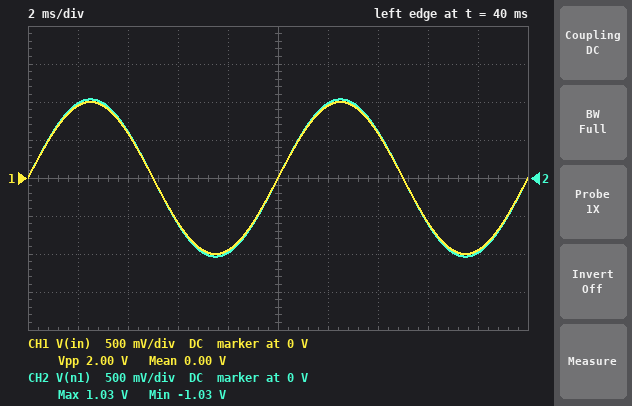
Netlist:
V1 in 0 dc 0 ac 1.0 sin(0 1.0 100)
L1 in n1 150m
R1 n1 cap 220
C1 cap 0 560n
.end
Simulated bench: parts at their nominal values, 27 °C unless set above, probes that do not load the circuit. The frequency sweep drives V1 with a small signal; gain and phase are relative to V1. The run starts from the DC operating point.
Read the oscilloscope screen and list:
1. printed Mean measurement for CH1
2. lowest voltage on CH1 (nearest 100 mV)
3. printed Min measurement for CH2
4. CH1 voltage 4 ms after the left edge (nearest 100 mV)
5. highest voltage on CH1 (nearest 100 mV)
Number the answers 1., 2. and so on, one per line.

1. 0.00 V
2. -1.0 V
3. -1.03 V
4. 600 mV
5. 1.0 V
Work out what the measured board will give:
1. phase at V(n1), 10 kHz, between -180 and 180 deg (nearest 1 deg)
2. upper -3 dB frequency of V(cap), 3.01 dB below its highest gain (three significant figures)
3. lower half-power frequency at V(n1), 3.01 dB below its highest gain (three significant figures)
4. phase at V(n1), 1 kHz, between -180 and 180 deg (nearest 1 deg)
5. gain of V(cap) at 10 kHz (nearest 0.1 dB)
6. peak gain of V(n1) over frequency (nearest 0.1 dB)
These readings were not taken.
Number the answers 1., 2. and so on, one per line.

1. -96 deg
2. 632 Hz
3. 396 Hz
4. -124 deg
5. -50.4 dB
6. 8.3 dB
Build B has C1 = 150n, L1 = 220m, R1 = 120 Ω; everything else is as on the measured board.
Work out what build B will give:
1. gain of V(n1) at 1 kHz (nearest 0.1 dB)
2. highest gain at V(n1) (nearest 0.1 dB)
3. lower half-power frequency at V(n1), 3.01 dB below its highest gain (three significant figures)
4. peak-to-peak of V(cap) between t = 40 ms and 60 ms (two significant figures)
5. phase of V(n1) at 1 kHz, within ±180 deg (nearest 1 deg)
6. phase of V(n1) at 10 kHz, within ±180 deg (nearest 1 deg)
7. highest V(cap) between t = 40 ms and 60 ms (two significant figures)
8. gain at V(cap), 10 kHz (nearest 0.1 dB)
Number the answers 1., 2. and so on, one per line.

1. 9.9 dB
2. 20.1 dB
3. 829 Hz
4. 2.0 V
5. -153 deg
6. -131 deg
7. 1.0 V
8. -42.2 dB
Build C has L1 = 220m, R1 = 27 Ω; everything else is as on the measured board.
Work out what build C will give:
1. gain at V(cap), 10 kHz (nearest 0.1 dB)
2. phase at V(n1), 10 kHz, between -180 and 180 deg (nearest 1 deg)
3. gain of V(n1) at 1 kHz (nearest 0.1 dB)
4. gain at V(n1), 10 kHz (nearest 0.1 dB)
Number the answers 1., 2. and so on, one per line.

1. -53.7 dB
2. -136 deg
3. -11.7 dB
4. -50.9 dB
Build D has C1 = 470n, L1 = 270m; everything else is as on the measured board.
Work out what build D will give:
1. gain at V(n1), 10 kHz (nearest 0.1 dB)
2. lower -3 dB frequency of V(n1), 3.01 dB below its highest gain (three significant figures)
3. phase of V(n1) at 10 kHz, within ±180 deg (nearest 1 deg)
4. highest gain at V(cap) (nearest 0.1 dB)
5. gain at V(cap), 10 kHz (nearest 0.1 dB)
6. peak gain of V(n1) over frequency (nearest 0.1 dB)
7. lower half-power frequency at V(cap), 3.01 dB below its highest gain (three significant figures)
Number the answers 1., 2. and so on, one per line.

1. -37.6 dB
2. 368 Hz
3. -98 deg
4. 10.8 dB
5. -54.0 dB
6. 11.2 dB
7. 366 Hz
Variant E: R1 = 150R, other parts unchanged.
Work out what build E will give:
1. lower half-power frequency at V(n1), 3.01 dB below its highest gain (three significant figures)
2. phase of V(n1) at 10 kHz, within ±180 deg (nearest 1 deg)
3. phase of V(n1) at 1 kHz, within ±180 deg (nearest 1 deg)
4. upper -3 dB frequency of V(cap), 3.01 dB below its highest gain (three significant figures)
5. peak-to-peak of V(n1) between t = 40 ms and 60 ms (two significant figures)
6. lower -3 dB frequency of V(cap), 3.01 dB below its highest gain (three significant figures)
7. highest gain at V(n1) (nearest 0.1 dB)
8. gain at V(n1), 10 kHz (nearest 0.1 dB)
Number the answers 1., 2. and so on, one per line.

1. 452 Hz
2. -100 deg
3. -139 deg
4. 613 Hz
5. 2.1 V
6. 450 Hz
7. 11.2 dB
8. -35.8 dB
